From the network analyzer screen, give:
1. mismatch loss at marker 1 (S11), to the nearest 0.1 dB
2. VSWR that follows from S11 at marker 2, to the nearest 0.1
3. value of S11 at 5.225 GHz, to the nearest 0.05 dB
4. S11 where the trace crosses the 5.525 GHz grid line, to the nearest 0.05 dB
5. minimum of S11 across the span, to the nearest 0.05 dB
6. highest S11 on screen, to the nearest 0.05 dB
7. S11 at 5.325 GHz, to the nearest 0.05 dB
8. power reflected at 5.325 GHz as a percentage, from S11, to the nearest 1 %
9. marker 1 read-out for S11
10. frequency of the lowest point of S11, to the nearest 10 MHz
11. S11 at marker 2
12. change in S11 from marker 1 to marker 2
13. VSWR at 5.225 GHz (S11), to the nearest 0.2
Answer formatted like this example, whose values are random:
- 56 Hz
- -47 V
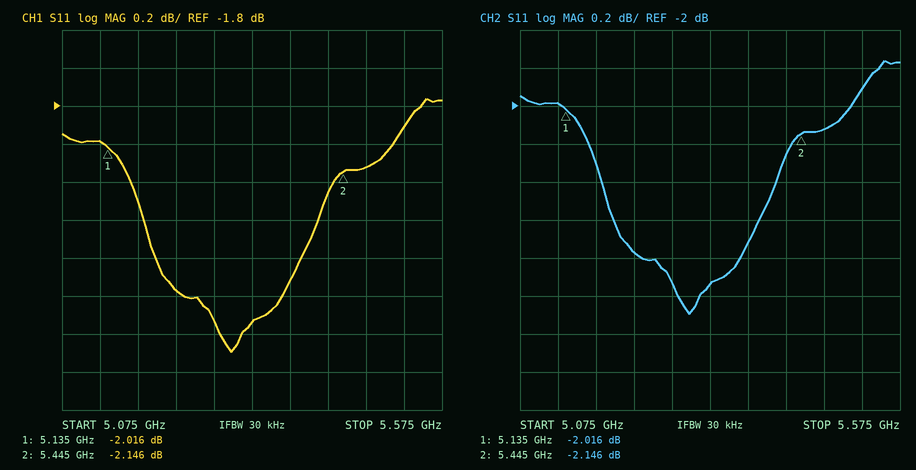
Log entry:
- 4.3 dB
- 8.1
- -2.75 dB
- -1.90 dB
- -3.10 dB
- -1.75 dB
- -2.95 dB
- 51 %
- -2.016 dB
- 5.30 GHz
- -2.146 dB
- -0.130 dB
- 6.4
